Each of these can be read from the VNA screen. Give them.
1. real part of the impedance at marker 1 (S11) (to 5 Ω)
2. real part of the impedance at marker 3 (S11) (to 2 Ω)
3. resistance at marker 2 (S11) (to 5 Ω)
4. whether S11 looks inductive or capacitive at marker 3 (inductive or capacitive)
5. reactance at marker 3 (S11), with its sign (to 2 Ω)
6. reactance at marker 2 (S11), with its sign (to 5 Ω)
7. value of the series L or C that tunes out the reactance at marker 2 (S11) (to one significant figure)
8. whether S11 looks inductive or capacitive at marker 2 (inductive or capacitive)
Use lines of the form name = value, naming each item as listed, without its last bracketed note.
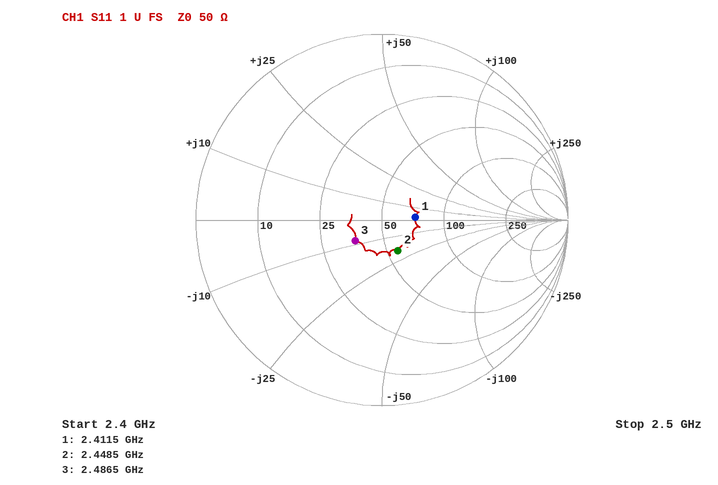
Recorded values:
real part of the impedance at marker 1 (S11) = 70 Ω
real part of the impedance at marker 3 (S11) = 36 Ω
resistance at marker 2 (S11) = 55 Ω
whether S11 looks inductive or capacitive at marker 3 = capacitive
reactance at marker 3 (S11), with its sign = -8 Ω
reactance at marker 2 (S11), with its sign = -20 Ω
value of the series L or C that tunes out the reactance at marker 2 (S11) = 1 nH
whether S11 looks inductive or capacitive at marker 2 = capacitive
